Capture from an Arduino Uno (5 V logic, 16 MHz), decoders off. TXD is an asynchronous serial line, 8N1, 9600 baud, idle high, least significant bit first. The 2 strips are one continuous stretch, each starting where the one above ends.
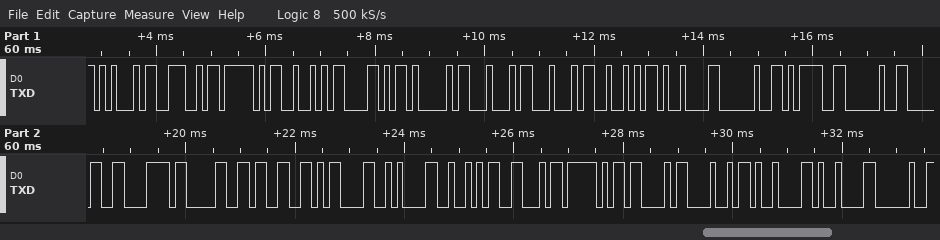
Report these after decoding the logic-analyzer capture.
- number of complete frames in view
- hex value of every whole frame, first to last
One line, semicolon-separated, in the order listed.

27; 45 4E 5F 52 58 41 44 44 52 09 20 3D 20 30 78 30 33 0D 0A 52 46 5F 43 48 09 09 20
